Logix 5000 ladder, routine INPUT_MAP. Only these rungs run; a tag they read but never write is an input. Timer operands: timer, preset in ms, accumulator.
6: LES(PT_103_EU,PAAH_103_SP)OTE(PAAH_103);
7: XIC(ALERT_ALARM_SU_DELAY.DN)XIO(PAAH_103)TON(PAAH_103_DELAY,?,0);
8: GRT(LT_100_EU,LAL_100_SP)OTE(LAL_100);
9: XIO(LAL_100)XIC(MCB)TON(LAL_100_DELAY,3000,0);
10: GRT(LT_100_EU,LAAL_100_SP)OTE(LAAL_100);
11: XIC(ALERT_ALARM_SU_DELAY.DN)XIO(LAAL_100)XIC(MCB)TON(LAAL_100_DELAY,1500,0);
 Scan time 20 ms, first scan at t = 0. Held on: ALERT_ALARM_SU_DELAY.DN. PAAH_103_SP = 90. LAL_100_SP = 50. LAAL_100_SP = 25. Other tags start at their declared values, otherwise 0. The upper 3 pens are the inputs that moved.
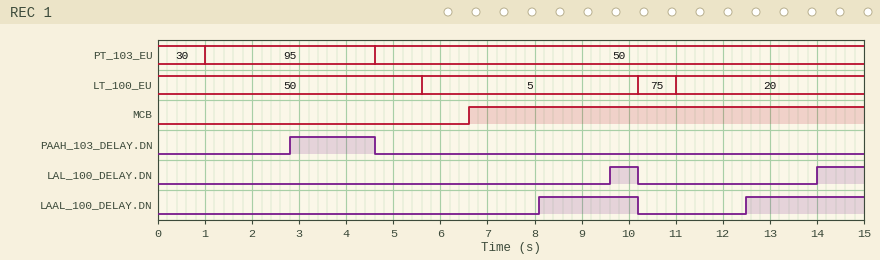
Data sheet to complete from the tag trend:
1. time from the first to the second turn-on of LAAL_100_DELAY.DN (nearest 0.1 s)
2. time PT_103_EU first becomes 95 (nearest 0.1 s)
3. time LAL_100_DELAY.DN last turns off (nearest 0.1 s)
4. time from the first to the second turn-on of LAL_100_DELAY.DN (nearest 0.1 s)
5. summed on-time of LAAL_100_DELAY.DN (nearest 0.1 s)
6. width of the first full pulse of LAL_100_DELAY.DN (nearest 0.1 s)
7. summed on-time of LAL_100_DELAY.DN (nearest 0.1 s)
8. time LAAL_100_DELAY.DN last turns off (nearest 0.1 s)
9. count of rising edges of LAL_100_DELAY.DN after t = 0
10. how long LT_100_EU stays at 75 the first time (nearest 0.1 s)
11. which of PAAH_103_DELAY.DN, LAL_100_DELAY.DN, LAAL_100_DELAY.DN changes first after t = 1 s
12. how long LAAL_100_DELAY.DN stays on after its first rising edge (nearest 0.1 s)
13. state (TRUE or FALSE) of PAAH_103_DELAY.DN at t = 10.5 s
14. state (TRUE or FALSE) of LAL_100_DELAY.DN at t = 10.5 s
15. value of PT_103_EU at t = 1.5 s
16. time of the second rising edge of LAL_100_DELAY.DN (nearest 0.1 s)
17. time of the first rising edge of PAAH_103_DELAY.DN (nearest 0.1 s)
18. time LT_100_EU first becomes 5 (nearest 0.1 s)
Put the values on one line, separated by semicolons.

4.4 s; 1.0 s; 10.2 s; 4.4 s; 4.6 s; 0.6 s; 1.6 s; 10.2 s; 2; 0.8 s; PAAH_103_DELAY.DN; 2.1 s; FALSE; FALSE; 95; 14.0 s; 2.8 s; 5.6 s
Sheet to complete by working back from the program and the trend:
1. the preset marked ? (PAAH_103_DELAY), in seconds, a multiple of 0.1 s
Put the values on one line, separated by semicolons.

1.8 s
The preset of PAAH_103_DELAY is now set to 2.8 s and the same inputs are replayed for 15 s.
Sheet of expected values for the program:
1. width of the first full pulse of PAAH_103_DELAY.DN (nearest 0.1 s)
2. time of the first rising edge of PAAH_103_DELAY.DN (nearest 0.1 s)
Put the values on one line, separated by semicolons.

0.8 s; 3.8 s
